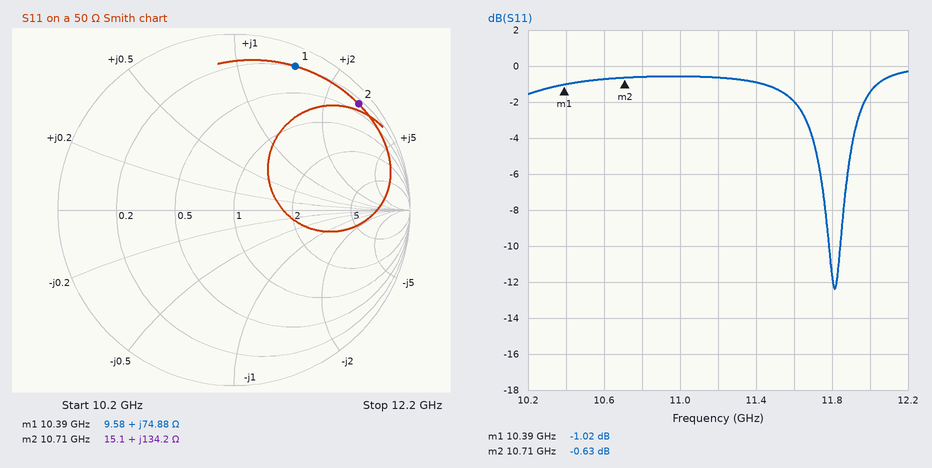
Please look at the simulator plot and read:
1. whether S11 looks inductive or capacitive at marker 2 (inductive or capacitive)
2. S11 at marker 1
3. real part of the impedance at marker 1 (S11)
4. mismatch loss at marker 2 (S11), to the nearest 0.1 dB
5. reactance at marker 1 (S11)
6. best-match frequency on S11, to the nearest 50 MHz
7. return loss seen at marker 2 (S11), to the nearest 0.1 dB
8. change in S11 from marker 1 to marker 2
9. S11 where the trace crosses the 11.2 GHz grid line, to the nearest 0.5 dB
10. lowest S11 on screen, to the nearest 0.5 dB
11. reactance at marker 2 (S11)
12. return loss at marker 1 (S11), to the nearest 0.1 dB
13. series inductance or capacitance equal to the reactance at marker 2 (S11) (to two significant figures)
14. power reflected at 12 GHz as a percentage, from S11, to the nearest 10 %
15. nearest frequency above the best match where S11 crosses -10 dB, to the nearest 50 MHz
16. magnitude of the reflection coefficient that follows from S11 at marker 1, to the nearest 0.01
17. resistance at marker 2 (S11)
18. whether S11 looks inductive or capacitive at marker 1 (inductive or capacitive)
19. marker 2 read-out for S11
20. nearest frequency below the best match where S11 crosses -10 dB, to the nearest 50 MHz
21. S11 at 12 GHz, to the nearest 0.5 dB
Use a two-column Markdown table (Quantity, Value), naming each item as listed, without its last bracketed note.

| Quantity | Value |
|---|---|
| whether S11 looks inductive or capacitive at marker 2 | inductive |
| S11 at marker 1 | -1.02 dB |
| real part of the impedance at marker 1 | 9.58 Ω |
| mismatch loss at marker 2 (S11), to the nearest 0.1 dB | 8.7 dB |
| reactance at marker 1 | +74.88 Ω |
| best-match frequency on S11, to the nearest 50 MHz | 11.80 GHz |
| return loss seen at marker 2 (S11), to the nearest 0.1 dB | 0.6 dB |
| change in S11 from marker 1 to marker 2 | 0.39 dB |
| S11 where the trace crosses the 11.2 GHz grid line, to the nearest 0.5 dB | -0.5 dB |
| lowest S11 on screen, to the nearest 0.5 dB | -12.5 dB |
| reactance at marker 2 | +134.2 Ω |
| return loss at marker 1 (S11), to the nearest 0.1 dB | 1.0 dB |
| series inductance or capacitance equal to the reactance at marker 2 (S11) | 2.0 nH |
| power reflected at 12 GHz as a percentage, from S11, to the nearest 10 % | 70 % |
| nearest frequency above the best match where S11 crosses -10 dB, to the nearest 50 MHz | 11.85 GHz |
| magnitude of the reflection coefficient that follows from S11 at marker 1, to the nearest 0.01 | 0.89 |
| resistance at marker 2 | 15.1 Ω |
| whether S11 looks inductive or capacitive at marker 1 | inductive |
| marker 2 read-out for S11 | -0.63 dB |
| nearest frequency below the best match where S11 crosses -10 dB, to the nearest 50 MHz | 11.80 GHz |
| S11 at 12 GHz, to the nearest 0.5 dB | -1.5 dB |
